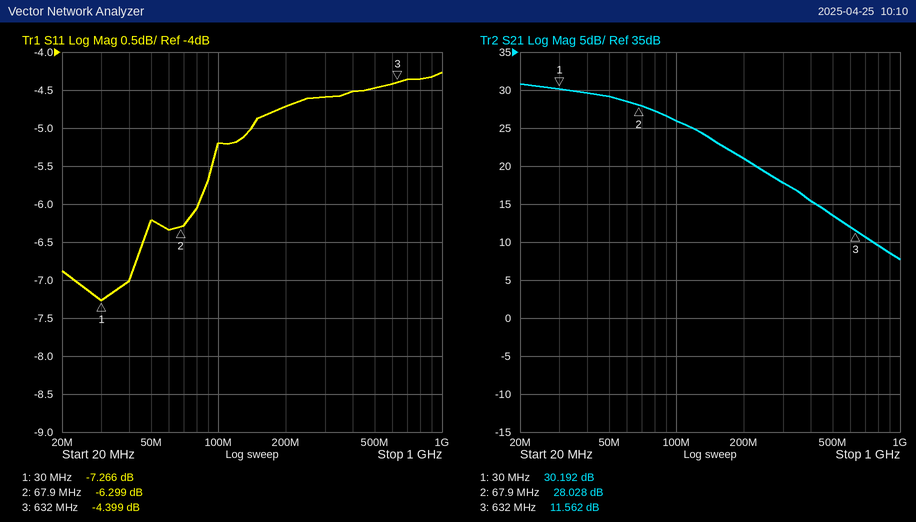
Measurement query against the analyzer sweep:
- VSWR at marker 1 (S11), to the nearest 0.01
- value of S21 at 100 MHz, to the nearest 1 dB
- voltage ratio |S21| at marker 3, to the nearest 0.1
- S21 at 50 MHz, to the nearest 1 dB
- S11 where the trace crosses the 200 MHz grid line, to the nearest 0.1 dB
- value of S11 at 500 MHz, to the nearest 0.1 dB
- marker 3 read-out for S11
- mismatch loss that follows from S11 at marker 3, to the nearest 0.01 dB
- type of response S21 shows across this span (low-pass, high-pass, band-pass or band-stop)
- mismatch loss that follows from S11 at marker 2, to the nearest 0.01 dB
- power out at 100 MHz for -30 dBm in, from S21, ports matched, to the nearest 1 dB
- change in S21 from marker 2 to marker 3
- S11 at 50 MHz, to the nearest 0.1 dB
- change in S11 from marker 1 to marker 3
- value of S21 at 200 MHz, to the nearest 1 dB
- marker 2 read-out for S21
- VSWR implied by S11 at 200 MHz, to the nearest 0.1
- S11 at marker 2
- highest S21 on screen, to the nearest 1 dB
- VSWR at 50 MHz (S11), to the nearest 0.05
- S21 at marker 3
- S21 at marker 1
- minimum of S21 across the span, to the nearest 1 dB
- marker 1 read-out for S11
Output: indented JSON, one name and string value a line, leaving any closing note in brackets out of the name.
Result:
{
  "VSWR at marker 1 (S11), to the nearest 0.01": "2.53",
  "value of S21 at 100 MHz, to the nearest 1 dB": "26 dB",
  "voltage ratio |S21| at marker 3, to the nearest 0.1": "3.8",
  "S21 at 50 MHz, to the nearest 1 dB": "29 dB",
  "S11 where the trace crosses the 200 MHz grid line, to the nearest 0.1 dB": "-4.7 dB",
  "value of S11 at 500 MHz, to the nearest 0.1 dB": "-4.5 dB",
  "marker 3 read-out for S11": "-4.399 dB",
  "mismatch loss that follows from S11 at marker 3, to the nearest 0.01 dB": "1.96 dB",
  "type of response S21 shows across this span": "low-pass",
  "mismatch loss that follows from S11 at marker 2, to the nearest 0.01 dB": "1.16 dB",
  "power out at 100 MHz for -30 dBm in, from S21, ports matched, to the nearest 1 dB": "-4 dBm",
  "change in S21 from marker 2 to marker 3": "-16.466 dB",
  "S11 at 50 MHz, to the nearest 0.1 dB": "-6.2 dB",
  "change in S11 from marker 1 to marker 3": "2.867 dB",
  "value of S21 at 200 MHz, to the nearest 1 dB": "21 dB",
  "marker 2 read-out for S21": "28.028 dB",
  "VSWR implied by S11 at 200 MHz, to the nearest 0.1": "3.8",
  "S11 at marker 2": "-6.299 dB",
  "highest S21 on screen, to the nearest 1 dB": "31 dB",
  "VSWR at 50 MHz (S11), to the nearest 0.05": "2.90",
  "S21 at marker 3": "11.562 dB",
  "S21 at marker 1": "30.192 dB",
  "minimum of S21 across the span, to the nearest 1 dB": "8 dB",
  "marker 1 read-out for S11": "-7.266 dB"
}
